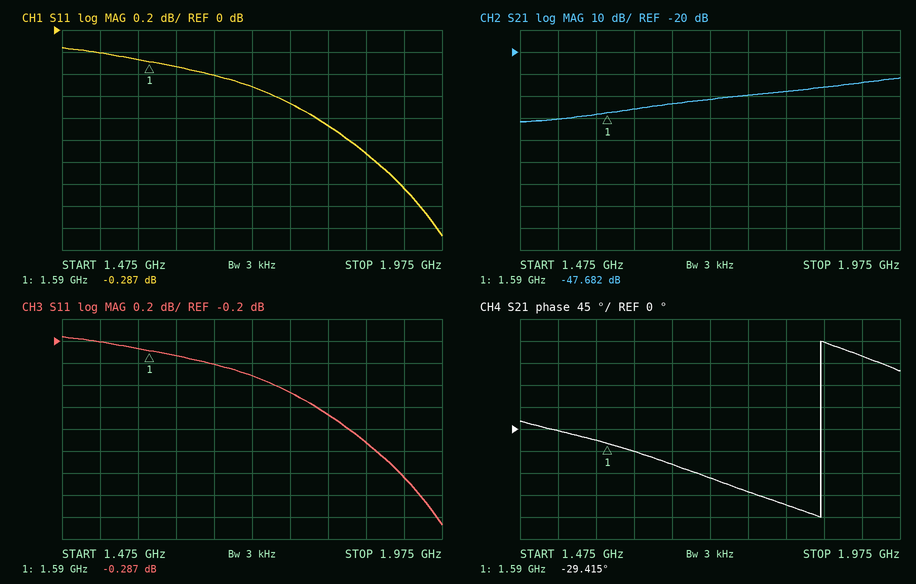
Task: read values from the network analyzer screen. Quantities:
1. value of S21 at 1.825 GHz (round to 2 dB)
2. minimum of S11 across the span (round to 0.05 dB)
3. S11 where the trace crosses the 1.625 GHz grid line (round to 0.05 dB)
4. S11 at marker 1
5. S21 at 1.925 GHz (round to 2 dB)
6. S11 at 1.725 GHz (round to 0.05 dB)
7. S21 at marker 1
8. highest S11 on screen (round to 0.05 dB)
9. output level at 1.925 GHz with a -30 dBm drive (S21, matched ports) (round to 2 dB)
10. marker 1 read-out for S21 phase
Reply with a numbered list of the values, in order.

1. -38 dB
2. -1.85 dB
3. -0.35 dB
4. -0.287 dB
5. -34 dB
6. -0.50 dB
7. -47.682 dB
8. -0.15 dB
9. -64 dBm
10. -29.415°
